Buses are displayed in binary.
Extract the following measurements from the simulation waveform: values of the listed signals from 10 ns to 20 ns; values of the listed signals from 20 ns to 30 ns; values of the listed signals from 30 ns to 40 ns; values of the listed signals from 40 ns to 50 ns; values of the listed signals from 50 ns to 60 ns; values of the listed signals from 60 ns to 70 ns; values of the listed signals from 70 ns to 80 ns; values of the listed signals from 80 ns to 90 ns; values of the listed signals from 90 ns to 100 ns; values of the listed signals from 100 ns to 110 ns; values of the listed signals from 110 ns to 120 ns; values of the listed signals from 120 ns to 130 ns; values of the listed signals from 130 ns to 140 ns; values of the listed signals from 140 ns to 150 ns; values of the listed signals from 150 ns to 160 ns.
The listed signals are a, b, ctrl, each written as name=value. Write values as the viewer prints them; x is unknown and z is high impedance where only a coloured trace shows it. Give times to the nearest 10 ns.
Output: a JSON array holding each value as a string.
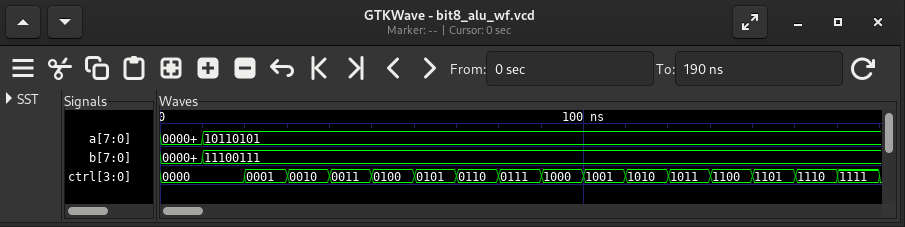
["a=10110101, b=11100111, ctrl=0000", "a=10110101, b=11100111, ctrl=0001", "a=10110101, b=11100111, ctrl=0010", "a=10110101, b=11100111, ctrl=0011", "a=10110101, b=11100111, ctrl=0100", "a=10110101, b=11100111, ctrl=0101", "a=10110101, b=11100111, ctrl=0110", "a=10110101, b=11100111, ctrl=0111", "a=10110101, b=11100111, ctrl=1000", "a=10110101, b=11100111, ctrl=1001", "a=10110101, b=11100111, ctrl=1010", "a=10110101, b=11100111, ctrl=1011", "a=10110101, b=11100111, ctrl=1100", "a=10110101, b=11100111, ctrl=1101", "a=10110101, b=11100111, ctrl=1110"]
